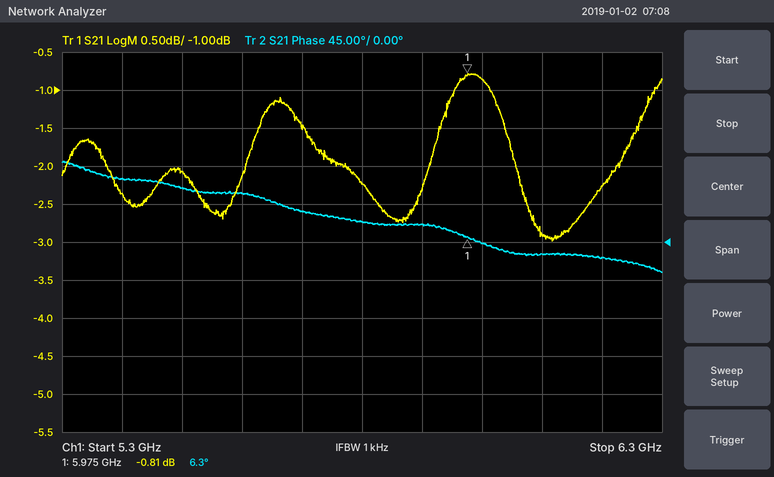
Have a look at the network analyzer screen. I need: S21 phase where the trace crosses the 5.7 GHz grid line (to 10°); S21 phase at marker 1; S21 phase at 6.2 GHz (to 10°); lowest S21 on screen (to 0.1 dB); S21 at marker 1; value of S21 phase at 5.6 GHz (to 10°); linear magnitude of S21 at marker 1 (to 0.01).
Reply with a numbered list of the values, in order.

1. 40°
2. 6.3°
3. -20°
4. -3.0 dB
5. -0.81 dB
6. 60°
7. 0.91
